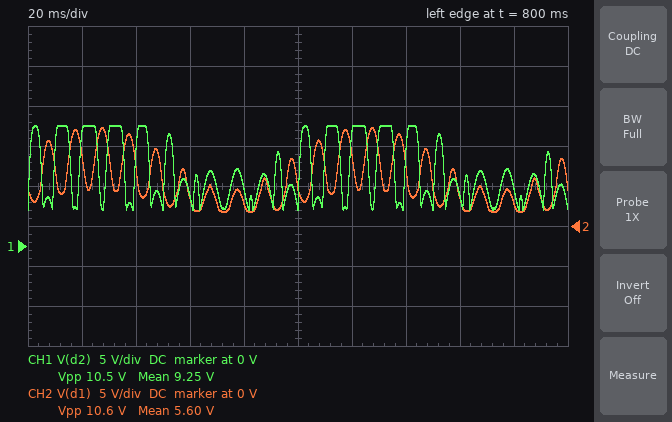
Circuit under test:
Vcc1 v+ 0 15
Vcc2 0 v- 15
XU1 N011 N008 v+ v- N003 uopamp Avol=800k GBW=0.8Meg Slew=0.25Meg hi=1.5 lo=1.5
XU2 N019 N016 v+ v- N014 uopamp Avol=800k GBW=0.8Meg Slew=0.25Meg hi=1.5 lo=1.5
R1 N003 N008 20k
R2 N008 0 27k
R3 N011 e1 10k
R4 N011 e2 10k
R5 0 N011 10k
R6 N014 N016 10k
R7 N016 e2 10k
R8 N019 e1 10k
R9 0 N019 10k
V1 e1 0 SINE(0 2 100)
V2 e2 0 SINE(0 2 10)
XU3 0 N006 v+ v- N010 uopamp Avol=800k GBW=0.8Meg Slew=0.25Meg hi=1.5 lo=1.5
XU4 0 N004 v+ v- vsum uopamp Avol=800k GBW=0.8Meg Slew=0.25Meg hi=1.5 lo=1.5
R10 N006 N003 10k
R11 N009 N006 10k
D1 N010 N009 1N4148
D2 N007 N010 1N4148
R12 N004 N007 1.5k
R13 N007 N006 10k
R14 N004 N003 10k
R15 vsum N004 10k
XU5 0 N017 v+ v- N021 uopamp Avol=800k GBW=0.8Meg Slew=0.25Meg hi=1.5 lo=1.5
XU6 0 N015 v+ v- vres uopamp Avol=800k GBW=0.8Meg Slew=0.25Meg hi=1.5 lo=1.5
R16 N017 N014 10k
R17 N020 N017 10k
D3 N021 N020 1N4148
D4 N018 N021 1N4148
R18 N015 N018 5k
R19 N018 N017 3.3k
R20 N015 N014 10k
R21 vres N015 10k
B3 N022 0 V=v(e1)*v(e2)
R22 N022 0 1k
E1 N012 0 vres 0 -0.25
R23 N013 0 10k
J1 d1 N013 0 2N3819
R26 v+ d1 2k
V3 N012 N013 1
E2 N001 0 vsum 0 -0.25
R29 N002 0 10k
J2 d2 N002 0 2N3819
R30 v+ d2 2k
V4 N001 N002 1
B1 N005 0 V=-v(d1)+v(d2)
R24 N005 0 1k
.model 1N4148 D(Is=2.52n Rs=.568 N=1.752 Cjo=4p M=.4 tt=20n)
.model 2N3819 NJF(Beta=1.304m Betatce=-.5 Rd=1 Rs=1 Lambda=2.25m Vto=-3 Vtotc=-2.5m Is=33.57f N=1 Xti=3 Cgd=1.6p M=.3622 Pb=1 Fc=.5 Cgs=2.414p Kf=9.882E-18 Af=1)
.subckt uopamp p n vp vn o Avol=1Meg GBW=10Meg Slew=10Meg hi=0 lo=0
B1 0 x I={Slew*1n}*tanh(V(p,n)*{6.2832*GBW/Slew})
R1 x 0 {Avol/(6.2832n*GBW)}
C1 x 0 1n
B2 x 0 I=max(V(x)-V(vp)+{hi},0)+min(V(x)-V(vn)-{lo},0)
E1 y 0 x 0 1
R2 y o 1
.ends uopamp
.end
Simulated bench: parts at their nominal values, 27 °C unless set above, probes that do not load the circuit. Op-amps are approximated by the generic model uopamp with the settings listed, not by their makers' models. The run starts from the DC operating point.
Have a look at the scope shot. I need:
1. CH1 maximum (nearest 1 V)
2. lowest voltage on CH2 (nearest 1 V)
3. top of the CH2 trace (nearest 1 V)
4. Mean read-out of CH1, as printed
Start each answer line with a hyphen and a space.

- 15 V
- 2 V
- 12 V
- 9.25 V
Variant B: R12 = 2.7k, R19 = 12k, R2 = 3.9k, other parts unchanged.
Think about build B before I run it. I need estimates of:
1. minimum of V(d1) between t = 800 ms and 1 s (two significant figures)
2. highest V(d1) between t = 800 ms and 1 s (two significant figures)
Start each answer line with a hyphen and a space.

- 4.5 V
- 14 V
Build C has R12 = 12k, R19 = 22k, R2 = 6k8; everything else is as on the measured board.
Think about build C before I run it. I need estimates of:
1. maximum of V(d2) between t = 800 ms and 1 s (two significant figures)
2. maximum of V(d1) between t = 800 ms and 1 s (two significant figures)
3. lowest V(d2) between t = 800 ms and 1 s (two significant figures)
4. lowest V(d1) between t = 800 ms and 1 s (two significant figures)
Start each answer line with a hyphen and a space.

- 14 V
- 15 V
- 2.2 V
- 4.5 V
